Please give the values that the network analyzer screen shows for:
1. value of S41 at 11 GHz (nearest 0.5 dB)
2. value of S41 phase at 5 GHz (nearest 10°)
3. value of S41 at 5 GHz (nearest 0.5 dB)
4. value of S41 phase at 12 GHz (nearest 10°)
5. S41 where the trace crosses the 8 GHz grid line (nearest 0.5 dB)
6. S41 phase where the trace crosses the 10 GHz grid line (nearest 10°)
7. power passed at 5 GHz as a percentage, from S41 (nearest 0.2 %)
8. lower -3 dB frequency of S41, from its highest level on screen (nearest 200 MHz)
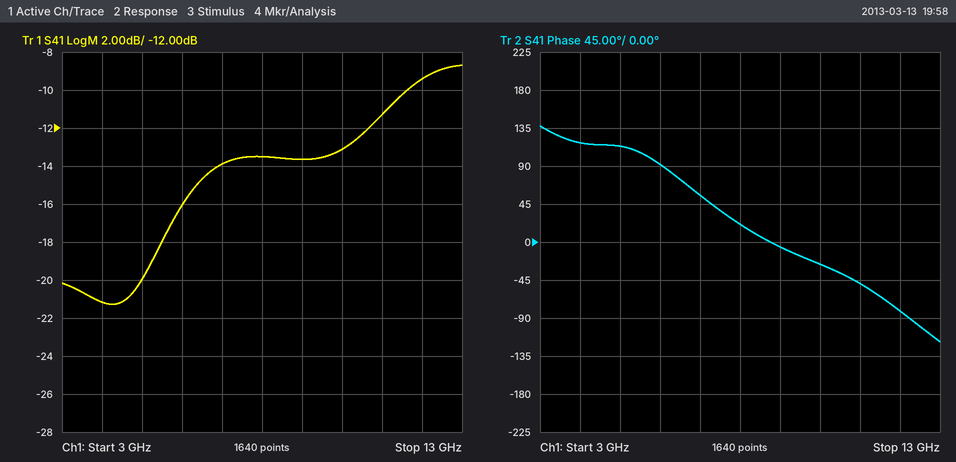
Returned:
-11.5 dB
110°
-20.0 dB
-80°
-13.5 dB
-30°
1.0 %
10.8 GHz
